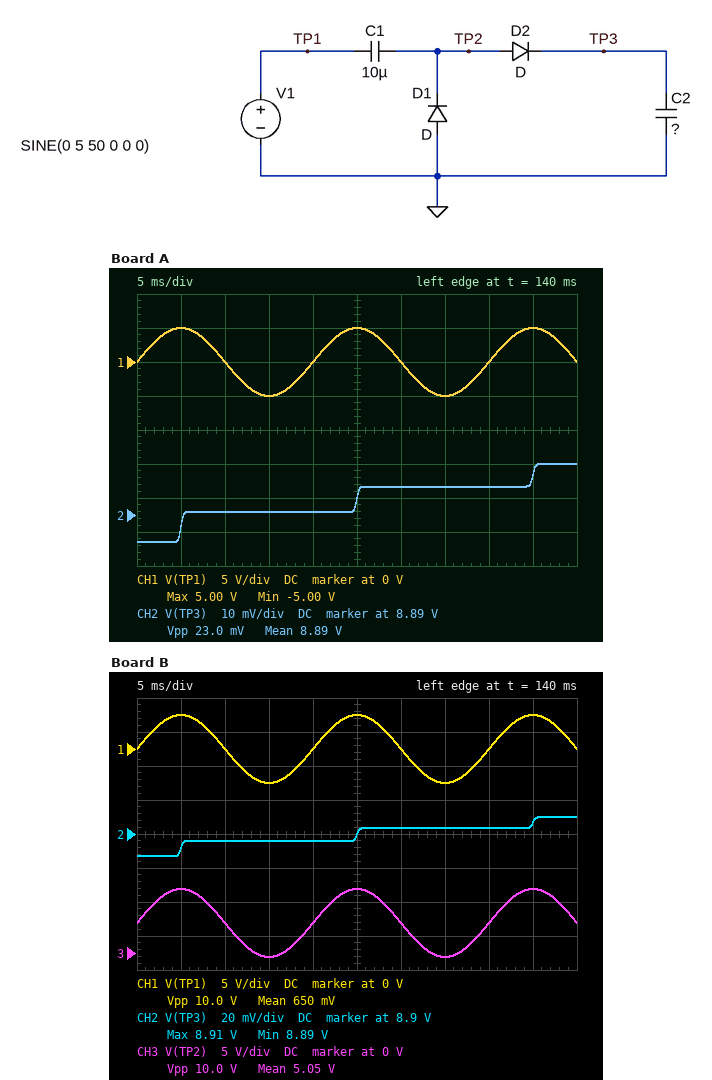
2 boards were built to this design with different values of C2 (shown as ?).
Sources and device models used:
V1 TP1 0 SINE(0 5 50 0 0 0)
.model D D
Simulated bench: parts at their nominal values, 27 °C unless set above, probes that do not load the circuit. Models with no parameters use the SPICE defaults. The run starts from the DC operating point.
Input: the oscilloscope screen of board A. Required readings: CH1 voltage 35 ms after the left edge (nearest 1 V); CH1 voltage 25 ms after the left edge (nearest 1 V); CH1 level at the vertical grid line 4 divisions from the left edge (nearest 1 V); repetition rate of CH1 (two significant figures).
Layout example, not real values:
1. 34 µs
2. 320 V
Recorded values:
1. -5 V
2. 5 V
3. 0 V
4. 50 Hz
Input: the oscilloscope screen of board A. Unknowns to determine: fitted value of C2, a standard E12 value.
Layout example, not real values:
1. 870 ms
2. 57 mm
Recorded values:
1. 390 nF
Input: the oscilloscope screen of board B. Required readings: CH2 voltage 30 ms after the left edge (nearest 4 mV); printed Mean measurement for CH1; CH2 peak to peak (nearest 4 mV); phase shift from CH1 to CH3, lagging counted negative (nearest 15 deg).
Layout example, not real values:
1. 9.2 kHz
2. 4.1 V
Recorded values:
1. 8.904 V
2. 650 mV
3. 24 mV
4. 0 deg
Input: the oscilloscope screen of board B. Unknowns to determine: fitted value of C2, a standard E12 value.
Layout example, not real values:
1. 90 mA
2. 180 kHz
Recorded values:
1. 330 nF
